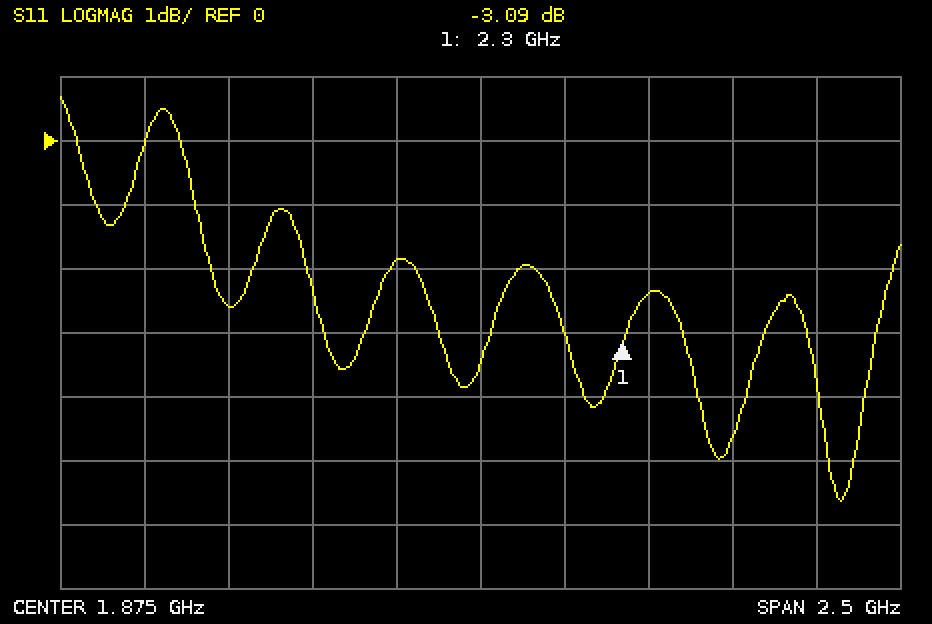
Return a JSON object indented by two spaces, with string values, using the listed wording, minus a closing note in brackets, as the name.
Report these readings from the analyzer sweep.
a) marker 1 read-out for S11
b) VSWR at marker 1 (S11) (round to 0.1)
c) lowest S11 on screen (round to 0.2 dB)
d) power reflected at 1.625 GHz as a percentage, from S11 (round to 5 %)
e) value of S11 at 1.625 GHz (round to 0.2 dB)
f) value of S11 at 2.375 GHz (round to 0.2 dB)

{
  "marker 1 read-out for S11": "-3.09 dB",
  "VSWR at marker 1 (S11)": "5.7",
  "lowest S11 on screen": "-5.6 dB",
  "power reflected at 1.625 GHz as a percentage, from S11": "65 %",
  "value of S11 at 1.625 GHz": "-1.8 dB",
  "value of S11 at 2.375 GHz": "-2.4 dB"
}
